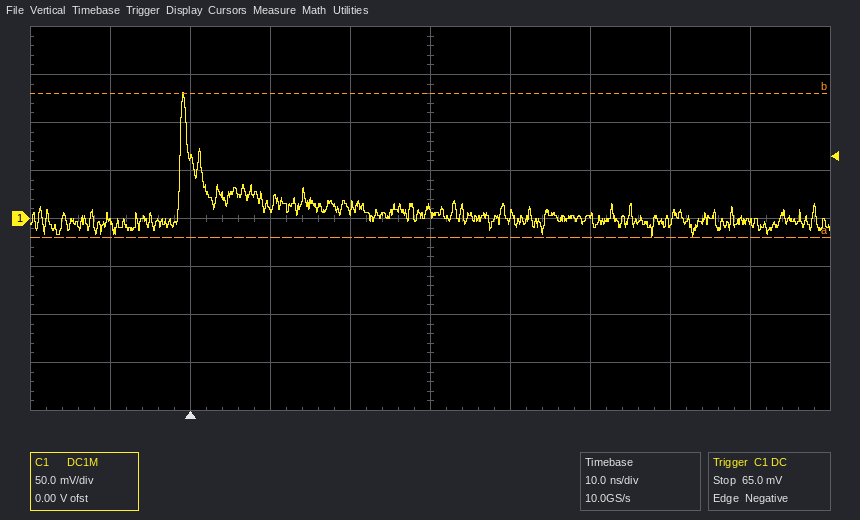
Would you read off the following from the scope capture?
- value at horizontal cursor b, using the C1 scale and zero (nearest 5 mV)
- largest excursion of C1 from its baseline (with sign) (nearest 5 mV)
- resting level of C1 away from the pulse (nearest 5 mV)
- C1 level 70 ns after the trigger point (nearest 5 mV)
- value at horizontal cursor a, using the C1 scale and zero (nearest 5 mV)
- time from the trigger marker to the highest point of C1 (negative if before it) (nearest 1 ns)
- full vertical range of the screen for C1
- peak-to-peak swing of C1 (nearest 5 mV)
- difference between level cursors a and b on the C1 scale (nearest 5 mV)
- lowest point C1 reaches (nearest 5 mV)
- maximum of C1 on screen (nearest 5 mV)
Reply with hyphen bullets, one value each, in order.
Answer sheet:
- 130 mV
- +130 mV
- 0 mV
- -5 mV
- -20 mV
- -1 ns
- 400 mV
- 150 mV
- 150 mV
- -20 mV
- 130 mV
